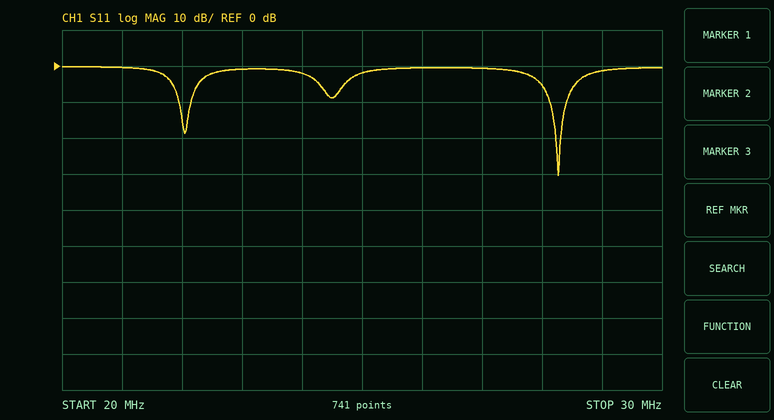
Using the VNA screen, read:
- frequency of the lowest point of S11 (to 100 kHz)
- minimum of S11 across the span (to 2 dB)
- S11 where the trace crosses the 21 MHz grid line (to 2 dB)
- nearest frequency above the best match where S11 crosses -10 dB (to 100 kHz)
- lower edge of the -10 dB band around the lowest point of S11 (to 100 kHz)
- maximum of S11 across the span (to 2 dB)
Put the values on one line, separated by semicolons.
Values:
28.3 MHz; -30 dB; 0 dB; 28.4 MHz; 28.1 MHz; 0 dB
